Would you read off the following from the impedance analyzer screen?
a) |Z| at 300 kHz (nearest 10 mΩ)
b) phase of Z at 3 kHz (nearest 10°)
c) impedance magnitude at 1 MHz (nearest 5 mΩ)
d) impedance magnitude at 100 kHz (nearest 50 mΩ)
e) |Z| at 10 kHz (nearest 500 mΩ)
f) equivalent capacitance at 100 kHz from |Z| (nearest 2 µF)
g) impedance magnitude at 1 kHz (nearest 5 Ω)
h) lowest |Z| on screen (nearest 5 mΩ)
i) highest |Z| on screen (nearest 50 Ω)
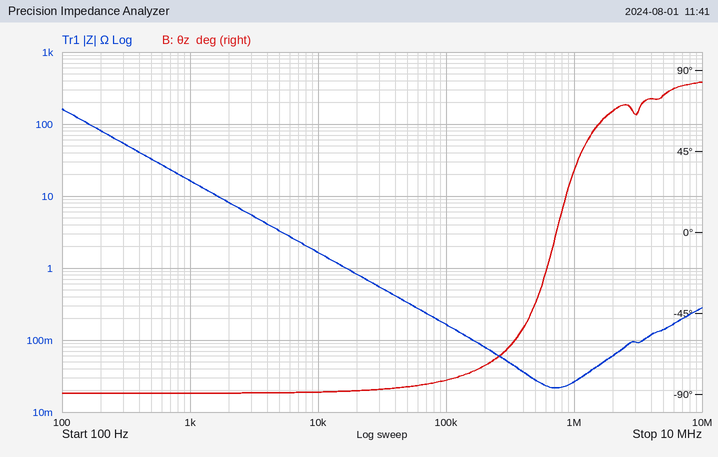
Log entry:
50 mΩ
-90°
25 mΩ
150 mΩ
1.5 Ω
10 µF
15 Ω
20 mΩ
150 Ω
